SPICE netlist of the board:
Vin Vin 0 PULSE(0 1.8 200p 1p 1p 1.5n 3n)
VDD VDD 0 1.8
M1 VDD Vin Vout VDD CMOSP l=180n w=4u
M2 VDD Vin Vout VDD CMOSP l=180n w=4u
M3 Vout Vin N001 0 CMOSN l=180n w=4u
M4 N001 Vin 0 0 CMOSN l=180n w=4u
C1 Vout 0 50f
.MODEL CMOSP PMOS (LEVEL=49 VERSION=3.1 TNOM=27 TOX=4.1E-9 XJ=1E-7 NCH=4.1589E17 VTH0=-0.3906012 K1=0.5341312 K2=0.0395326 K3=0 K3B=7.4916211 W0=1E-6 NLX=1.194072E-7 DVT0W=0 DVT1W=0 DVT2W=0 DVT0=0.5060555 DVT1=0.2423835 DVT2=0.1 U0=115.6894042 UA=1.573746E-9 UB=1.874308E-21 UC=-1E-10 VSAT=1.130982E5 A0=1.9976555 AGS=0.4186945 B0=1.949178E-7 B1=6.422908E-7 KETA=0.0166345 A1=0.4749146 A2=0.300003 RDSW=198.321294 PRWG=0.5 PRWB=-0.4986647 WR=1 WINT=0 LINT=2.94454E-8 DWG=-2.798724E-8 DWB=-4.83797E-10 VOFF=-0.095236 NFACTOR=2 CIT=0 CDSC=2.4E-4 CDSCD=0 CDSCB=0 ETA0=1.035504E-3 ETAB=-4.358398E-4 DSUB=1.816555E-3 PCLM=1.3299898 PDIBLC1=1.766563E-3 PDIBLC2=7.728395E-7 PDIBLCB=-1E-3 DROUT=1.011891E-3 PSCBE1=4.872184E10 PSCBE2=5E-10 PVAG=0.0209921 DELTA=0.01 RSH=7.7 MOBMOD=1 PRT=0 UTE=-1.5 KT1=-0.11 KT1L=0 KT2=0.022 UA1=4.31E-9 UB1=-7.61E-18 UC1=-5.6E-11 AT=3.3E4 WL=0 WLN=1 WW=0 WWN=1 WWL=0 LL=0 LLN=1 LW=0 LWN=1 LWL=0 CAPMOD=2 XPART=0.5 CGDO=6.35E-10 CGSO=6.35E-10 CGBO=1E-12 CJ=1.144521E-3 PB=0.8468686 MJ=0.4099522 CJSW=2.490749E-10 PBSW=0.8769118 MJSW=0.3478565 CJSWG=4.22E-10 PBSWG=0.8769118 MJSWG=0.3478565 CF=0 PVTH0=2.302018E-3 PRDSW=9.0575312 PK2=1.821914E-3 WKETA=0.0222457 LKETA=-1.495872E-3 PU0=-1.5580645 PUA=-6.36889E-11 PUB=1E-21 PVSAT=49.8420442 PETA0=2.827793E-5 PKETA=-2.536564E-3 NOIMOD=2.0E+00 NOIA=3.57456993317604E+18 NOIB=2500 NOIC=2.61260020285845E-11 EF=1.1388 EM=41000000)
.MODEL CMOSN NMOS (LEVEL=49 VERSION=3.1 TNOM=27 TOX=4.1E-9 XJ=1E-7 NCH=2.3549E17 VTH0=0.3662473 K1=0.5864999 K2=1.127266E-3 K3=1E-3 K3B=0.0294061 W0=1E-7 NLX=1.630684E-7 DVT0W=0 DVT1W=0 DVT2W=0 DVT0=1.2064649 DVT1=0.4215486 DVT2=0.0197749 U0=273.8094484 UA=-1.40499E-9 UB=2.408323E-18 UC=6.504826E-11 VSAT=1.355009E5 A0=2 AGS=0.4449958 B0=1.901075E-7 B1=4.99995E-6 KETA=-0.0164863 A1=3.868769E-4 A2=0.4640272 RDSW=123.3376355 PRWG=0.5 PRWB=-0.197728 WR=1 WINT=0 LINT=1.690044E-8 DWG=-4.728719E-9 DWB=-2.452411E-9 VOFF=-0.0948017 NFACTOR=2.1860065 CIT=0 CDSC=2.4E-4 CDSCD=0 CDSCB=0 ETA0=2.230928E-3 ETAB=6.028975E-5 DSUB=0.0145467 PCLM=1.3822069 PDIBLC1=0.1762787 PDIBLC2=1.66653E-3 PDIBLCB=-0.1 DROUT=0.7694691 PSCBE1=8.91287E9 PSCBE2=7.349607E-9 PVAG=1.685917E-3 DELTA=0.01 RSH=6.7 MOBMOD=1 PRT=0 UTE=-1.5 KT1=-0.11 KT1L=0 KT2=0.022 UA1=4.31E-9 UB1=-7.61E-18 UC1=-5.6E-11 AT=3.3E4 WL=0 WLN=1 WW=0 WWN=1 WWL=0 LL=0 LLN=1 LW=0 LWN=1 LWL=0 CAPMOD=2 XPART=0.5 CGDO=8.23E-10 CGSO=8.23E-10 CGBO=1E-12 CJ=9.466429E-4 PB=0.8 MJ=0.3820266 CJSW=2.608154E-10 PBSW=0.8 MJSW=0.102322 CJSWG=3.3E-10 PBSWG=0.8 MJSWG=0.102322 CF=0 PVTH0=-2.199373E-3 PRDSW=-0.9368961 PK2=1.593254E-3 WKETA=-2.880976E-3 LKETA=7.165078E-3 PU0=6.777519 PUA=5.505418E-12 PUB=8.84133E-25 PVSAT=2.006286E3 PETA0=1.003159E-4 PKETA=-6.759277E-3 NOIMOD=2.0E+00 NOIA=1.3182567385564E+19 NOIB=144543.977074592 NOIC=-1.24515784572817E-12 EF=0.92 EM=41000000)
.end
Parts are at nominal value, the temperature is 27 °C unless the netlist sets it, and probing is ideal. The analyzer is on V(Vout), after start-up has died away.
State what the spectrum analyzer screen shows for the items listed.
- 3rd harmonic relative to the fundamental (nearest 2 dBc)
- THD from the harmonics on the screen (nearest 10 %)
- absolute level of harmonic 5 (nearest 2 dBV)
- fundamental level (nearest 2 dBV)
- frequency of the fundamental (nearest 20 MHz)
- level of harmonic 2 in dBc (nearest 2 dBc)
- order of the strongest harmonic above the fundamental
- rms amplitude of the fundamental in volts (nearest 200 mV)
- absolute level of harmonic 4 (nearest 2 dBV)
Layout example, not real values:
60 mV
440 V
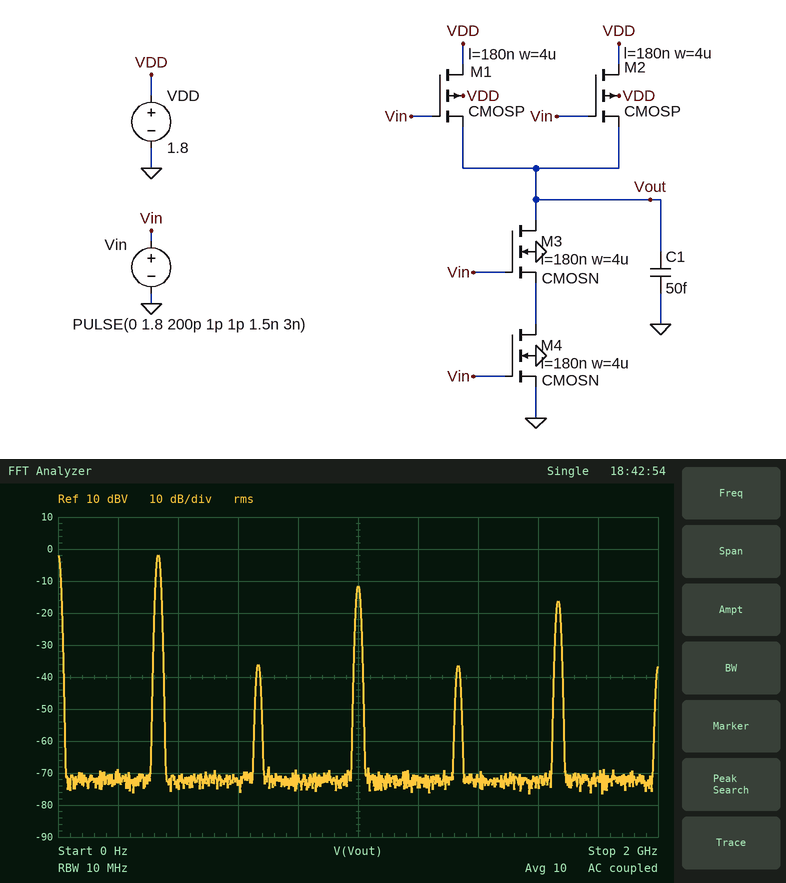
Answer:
-10 dBc
40 %
-16 dBV
-2 dBV
340 MHz
-34 dBc
3
800 mV
-36 dBV
